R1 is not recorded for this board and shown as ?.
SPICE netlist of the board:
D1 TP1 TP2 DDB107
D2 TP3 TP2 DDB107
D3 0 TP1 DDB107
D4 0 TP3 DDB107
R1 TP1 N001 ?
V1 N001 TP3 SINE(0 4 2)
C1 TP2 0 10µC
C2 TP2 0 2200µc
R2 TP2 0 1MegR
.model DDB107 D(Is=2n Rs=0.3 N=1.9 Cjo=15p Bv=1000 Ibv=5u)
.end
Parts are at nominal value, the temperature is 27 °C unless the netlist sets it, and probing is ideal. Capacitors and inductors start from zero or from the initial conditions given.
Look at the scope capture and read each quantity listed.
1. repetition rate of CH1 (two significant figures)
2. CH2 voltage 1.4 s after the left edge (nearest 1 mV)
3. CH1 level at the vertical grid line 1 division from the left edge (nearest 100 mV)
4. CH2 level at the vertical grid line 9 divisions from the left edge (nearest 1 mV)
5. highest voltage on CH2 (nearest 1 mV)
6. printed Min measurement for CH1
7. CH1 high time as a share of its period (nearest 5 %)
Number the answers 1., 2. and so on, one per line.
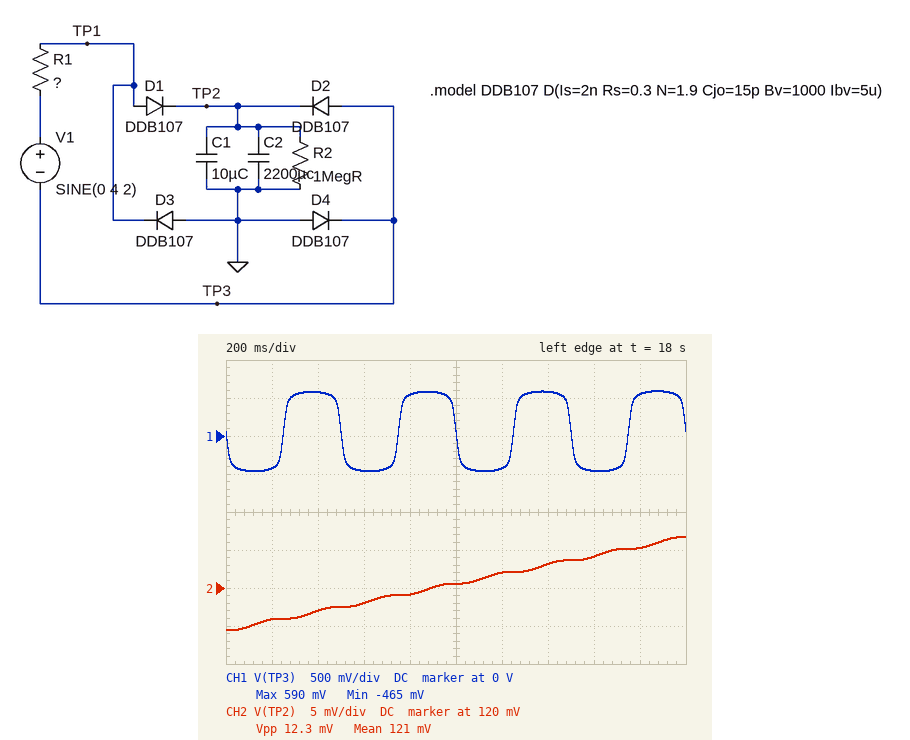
1. 2.0 Hz
2. 123 mV
3. -400 mV
4. 125 mV
5. 127 mV
6. -465 mV
7. 50 %
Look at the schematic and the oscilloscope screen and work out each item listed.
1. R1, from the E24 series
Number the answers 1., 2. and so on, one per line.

1. 120 kΩ
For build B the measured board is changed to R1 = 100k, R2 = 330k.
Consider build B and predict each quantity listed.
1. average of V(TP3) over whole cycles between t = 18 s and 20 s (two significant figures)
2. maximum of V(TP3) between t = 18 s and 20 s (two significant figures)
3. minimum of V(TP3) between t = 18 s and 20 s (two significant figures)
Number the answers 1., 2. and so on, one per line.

1. 71 mV
2. 620 mV
3. -470 mV
